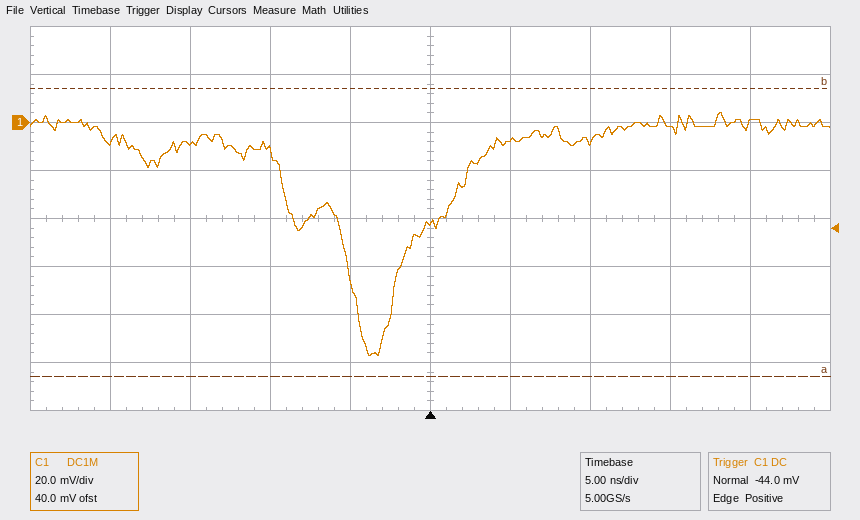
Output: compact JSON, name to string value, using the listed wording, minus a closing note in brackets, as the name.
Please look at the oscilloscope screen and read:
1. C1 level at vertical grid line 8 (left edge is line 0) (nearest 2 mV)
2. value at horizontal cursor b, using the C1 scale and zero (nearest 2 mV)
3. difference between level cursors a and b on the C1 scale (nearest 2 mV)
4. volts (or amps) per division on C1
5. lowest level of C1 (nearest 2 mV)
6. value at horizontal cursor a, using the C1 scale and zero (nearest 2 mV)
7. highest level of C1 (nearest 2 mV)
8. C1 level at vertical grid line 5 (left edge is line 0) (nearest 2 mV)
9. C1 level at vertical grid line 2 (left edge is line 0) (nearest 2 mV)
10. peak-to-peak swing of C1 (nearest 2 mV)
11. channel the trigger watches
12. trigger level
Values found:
{"C1 level at vertical grid line 8 (left edge is line 0)": "-2 mV", "value at horizontal cursor b, using the C1 scale and zero": "14 mV", "difference between level cursors a and b on the C1 scale": "120 mV", "volts (or amps) per division on C1": "20 mV", "lowest level of C1": "-98 mV", "value at horizontal cursor a, using the C1 scale and zero": "-106 mV", "highest level of C1": "4 mV", "C1 level at vertical grid line 5 (left edge is line 0)": "-42 mV", "C1 level at vertical grid line 2 (left edge is line 0)": "-8 mV", "peak-to-peak swing of C1": "102 mV", "channel the trigger watches": "C1", "trigger level": "-44.0 mV"}
